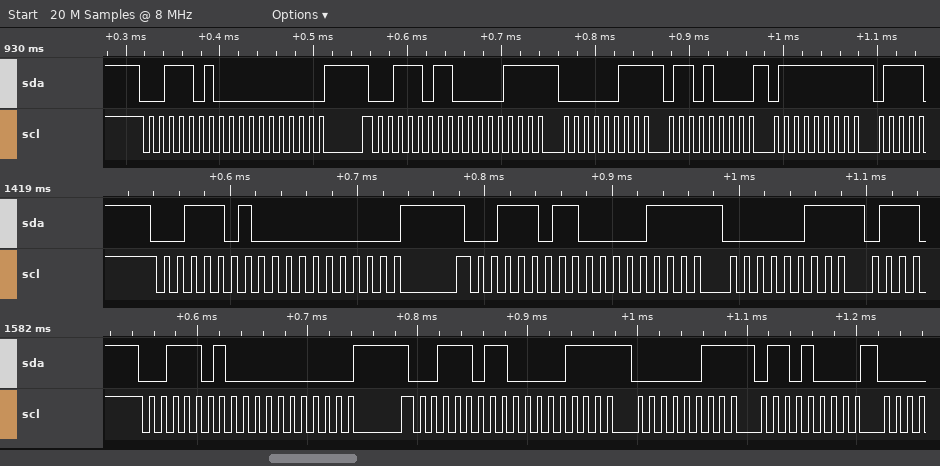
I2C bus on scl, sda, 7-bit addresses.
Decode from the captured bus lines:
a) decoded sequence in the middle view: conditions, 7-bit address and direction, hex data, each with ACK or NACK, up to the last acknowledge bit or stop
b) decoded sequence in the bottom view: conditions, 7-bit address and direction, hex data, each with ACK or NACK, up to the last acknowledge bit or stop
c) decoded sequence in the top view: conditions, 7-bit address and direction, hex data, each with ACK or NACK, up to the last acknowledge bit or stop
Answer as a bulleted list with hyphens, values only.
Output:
- start, address 1D write ACK, 00 ACK, repeated start, address 1D read ACK, 0F ACK, 07 ACK
- start, address 1D write ACK, 00 ACK, repeated start, address 1D read ACK, 0F ACK, 07 ACK, D0 ACK
- start, address 1D write ACK, 00 ACK, repeated start, address 1D read ACK, 0F ACK, 07 ACK, D0 ACK, FF ACK
